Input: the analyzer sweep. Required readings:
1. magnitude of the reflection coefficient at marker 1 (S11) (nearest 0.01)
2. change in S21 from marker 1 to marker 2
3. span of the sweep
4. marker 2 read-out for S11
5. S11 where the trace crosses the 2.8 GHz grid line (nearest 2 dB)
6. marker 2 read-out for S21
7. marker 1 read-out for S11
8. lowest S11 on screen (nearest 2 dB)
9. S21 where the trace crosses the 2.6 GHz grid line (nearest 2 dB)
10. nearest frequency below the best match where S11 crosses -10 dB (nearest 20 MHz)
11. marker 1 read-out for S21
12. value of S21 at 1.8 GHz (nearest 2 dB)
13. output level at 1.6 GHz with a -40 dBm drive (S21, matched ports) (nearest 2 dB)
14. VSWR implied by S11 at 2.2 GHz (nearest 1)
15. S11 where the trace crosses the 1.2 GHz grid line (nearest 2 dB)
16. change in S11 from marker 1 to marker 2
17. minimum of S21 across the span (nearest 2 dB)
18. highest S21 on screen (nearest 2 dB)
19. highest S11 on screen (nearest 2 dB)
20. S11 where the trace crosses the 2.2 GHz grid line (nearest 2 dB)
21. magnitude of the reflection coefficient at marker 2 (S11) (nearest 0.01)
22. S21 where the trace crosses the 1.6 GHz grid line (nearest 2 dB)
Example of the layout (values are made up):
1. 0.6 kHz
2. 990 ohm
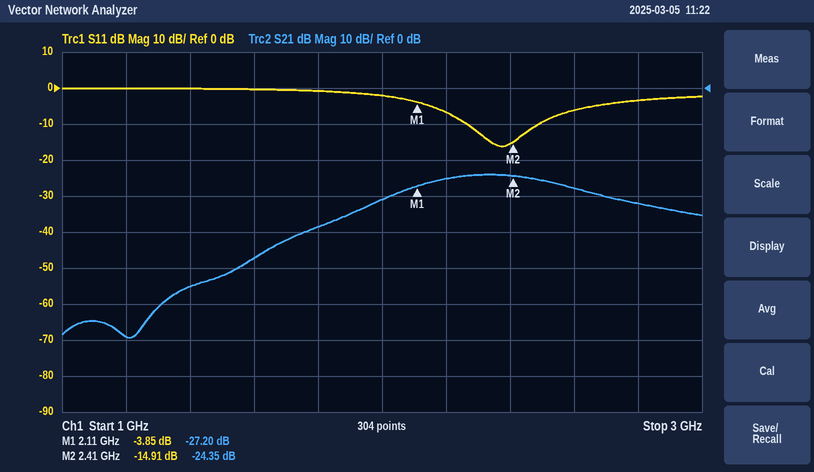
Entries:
1. 0.64
2. 2.85 dB
3. 2 GHz
4. -14.91 dB
5. -4 dB
6. -24.35 dB
7. -3.85 dB
8. -16 dB
9. -28 dB
10. 2.26 GHz
11. -27.20 dB
12. -38 dB
13. -88 dBm
14. 3
15. 0 dB
16. -11.06 dB
17. -70 dB
18. -24 dB
19. 0 dB
20. -6 dB
21. 0.18
22. -48 dB
